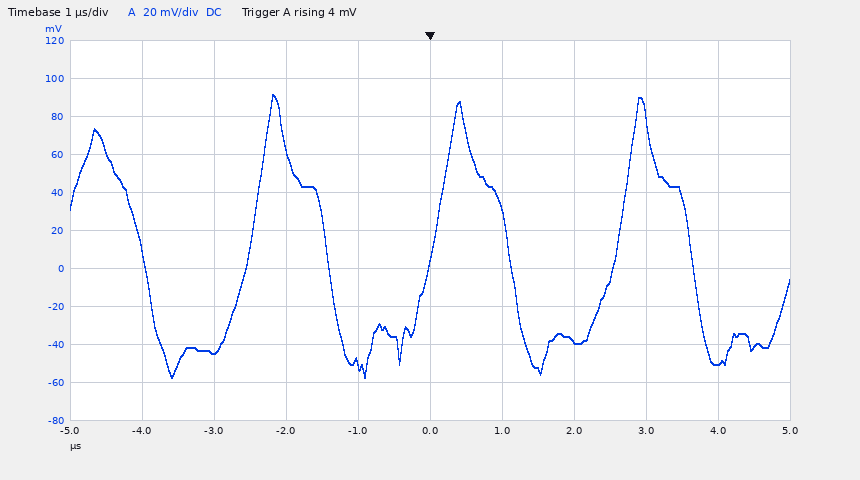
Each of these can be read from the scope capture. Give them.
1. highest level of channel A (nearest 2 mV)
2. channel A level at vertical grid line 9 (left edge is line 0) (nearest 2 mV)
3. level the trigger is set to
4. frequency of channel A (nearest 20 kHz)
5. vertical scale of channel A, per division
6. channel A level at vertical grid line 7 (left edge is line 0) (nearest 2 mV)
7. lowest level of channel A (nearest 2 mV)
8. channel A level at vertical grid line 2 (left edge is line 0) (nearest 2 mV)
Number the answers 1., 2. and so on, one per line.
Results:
1. 92 mV
2. -50 mV
3. 4 mV
4. 400 kHz
5. 20 mV
6. -38 mV
7. -58 mV
8. -44 mV
